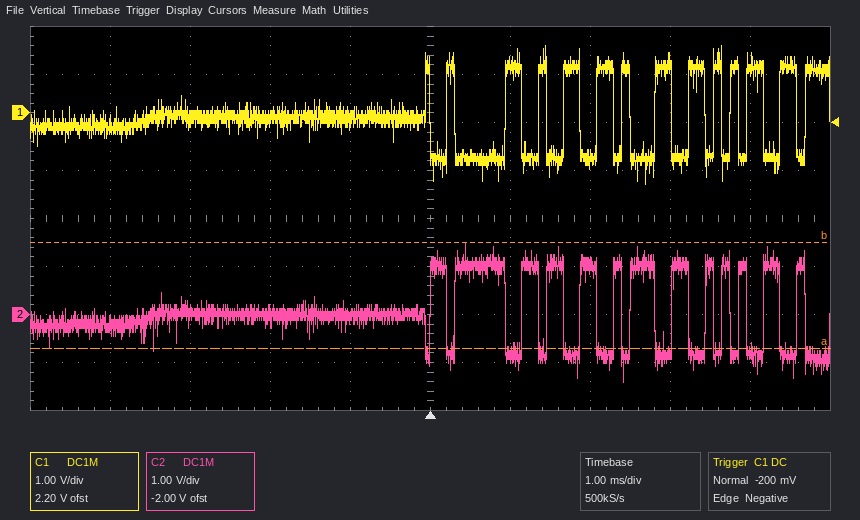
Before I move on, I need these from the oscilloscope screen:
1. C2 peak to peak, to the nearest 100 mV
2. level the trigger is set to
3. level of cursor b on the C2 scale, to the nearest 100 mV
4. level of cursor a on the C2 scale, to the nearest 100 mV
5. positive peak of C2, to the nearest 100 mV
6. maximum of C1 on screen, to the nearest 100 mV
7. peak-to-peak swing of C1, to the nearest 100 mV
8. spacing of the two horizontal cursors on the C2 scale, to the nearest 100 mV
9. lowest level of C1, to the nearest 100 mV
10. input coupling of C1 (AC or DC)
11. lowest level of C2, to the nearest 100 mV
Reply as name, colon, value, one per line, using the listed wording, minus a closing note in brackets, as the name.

C2 peak to peak, to the nearest 100 mV: 2.9 V
level the trigger is set to: -200 mV
level of cursor b on the C2 scale, to the nearest 100 mV: 1.5 V
level of cursor a on the C2 scale, to the nearest 100 mV: -700 mV
positive peak of C2, to the nearest 100 mV: 1.5 V
maximum of C1 on screen, to the nearest 100 mV: 1.4 V
peak-to-peak swing of C1, to the nearest 100 mV: 2.9 V
spacing of the two horizontal cursors on the C2 scale, to the nearest 100 mV: 2.2 V
lowest level of C1, to the nearest 100 mV: -1.5 V
input coupling of C1: DC
lowest level of C2, to the nearest 100 mV: -1.4 V
